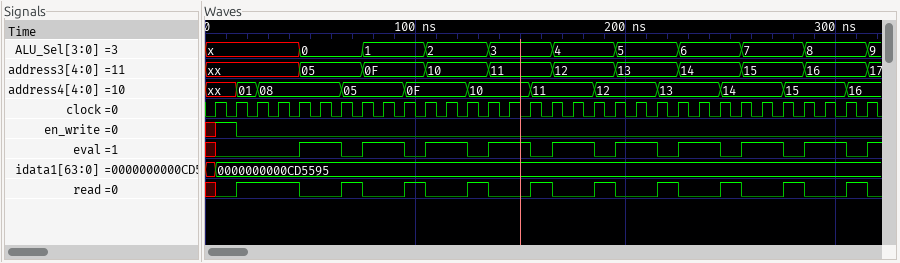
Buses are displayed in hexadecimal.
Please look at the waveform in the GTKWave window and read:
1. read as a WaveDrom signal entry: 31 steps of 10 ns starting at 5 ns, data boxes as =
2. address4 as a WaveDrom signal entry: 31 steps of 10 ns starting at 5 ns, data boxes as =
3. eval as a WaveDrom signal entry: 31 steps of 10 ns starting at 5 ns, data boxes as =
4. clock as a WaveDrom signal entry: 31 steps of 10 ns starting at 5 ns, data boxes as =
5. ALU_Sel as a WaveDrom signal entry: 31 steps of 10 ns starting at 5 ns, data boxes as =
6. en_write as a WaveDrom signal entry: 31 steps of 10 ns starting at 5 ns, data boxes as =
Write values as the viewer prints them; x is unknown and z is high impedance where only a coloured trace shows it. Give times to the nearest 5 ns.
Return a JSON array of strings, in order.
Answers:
["{name: 'read', wave: '01..0.10.10.10.10.10.10.10.10.1'}", "{name: 'address4', wave: 'x==...=..=..=..=..=..=..=..=..=', data: '01 08 05 0F 10 11 12 13 14 15 16'}", "{name: 'eval', wave: '0...1.01.01.01.01.01.01.01.01.0'}", "{name: 'clock', wave: 'p..............................'}", "{name: 'ALU_Sel', wave: 'x...=..=..=..=..=..=..=..=..=..', data: '0 1 2 3 4 5 6 7 8'}", "{name: 'en_write', wave: '10.............................'}"]
